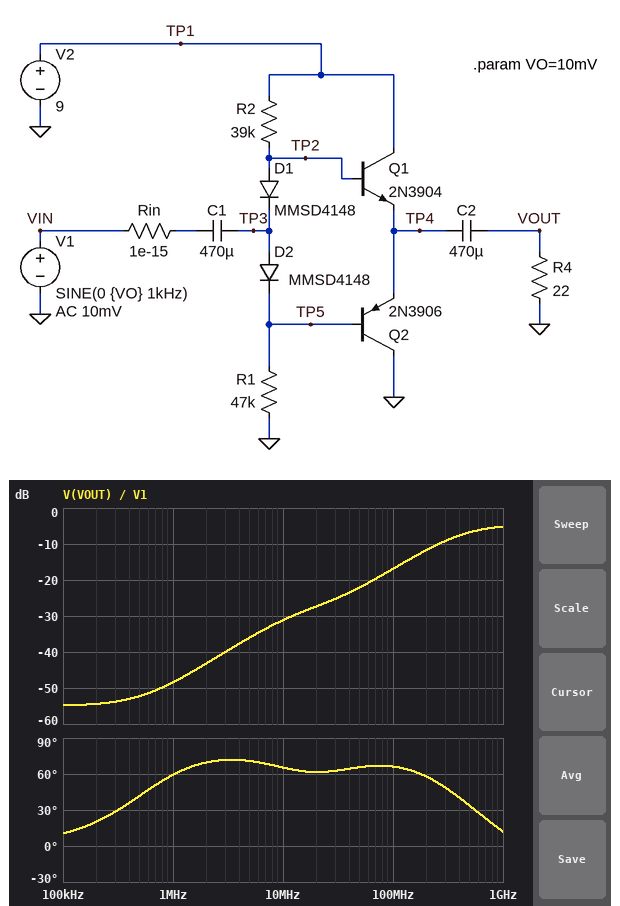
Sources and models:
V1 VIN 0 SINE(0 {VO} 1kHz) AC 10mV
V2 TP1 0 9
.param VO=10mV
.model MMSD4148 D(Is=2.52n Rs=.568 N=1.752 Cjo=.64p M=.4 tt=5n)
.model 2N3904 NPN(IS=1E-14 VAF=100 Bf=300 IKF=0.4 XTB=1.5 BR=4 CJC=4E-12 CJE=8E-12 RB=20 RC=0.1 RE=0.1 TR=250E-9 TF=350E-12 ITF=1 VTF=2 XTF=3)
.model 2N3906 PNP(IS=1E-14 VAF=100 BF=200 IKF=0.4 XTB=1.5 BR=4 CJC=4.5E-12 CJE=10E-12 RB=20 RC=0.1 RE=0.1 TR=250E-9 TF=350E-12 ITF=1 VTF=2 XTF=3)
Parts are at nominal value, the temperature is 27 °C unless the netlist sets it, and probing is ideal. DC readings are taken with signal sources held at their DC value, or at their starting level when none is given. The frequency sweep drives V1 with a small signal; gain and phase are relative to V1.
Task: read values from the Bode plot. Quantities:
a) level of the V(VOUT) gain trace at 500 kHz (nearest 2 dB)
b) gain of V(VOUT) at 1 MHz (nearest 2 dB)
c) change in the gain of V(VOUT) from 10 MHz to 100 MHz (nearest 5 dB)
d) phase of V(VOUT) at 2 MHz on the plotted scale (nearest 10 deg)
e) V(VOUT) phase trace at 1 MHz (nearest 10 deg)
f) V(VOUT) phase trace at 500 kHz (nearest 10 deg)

-52 dB
-48 dB
15 dB
70 deg
60 deg
40 deg
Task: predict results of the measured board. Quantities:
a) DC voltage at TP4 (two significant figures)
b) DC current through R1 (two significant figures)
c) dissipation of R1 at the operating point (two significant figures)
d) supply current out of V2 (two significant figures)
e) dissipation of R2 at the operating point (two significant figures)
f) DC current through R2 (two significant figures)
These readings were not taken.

4.9 V
94 µA
410 µW
95 µA
340 µW
94 µA
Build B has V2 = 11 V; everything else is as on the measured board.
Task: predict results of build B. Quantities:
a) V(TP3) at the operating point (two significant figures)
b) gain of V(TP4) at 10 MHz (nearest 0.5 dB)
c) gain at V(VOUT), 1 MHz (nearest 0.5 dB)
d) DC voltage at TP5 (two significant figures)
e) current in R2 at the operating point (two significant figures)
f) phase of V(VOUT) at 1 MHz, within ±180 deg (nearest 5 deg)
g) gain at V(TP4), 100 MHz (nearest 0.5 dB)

6.0 V
-30.5 dB
-47.5 dB
5.5 V
120 µA
50 deg
-16.0 dB
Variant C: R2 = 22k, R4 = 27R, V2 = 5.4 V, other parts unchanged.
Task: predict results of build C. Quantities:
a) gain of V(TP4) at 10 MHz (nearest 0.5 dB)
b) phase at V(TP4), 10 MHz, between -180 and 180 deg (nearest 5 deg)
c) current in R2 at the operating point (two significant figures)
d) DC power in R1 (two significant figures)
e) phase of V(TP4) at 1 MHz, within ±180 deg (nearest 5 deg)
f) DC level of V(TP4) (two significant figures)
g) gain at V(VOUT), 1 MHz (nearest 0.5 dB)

-30.5 dB
60 deg
65 µA
200 µW
70 deg
3.5 V
-47.5 dB
